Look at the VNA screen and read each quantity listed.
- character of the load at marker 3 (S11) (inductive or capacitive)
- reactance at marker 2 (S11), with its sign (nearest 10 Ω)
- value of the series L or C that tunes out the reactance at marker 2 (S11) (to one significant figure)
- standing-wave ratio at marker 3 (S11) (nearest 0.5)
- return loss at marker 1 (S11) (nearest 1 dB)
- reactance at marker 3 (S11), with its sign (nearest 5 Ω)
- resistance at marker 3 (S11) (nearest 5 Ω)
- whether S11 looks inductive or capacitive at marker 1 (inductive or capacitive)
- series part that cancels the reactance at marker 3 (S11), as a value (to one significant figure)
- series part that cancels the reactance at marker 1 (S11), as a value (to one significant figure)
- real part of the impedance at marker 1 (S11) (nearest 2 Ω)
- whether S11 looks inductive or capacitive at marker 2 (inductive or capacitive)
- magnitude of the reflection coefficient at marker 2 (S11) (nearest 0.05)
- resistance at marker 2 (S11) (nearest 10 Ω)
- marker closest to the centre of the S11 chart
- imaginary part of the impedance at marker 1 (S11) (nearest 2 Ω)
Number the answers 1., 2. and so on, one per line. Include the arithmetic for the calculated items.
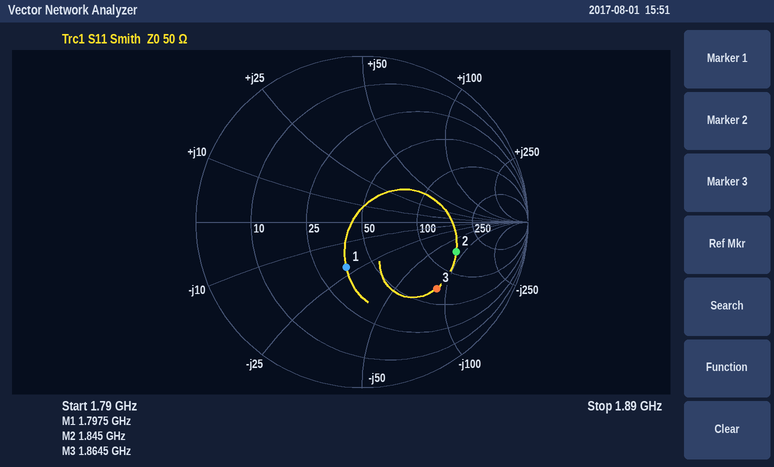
1. capacitive
2. -80 Ω
3. L = 80 Ω/(2π × 1.845 GHz) ≈ 7 nH
4. 4.0
5. 11 dB
6. -85 Ω
7. 70 Ω
8. capacitive
9. L = 85 Ω/(2π × 1.8645 GHz) ≈ 7 nH
10. L = 22 Ω/(2π × 1.7975 GHz) ≈ 2 nH
11. 36 Ω
12. capacitive
13. 0.60
14. 150 Ω
15. marker 1
16. -22 Ω
